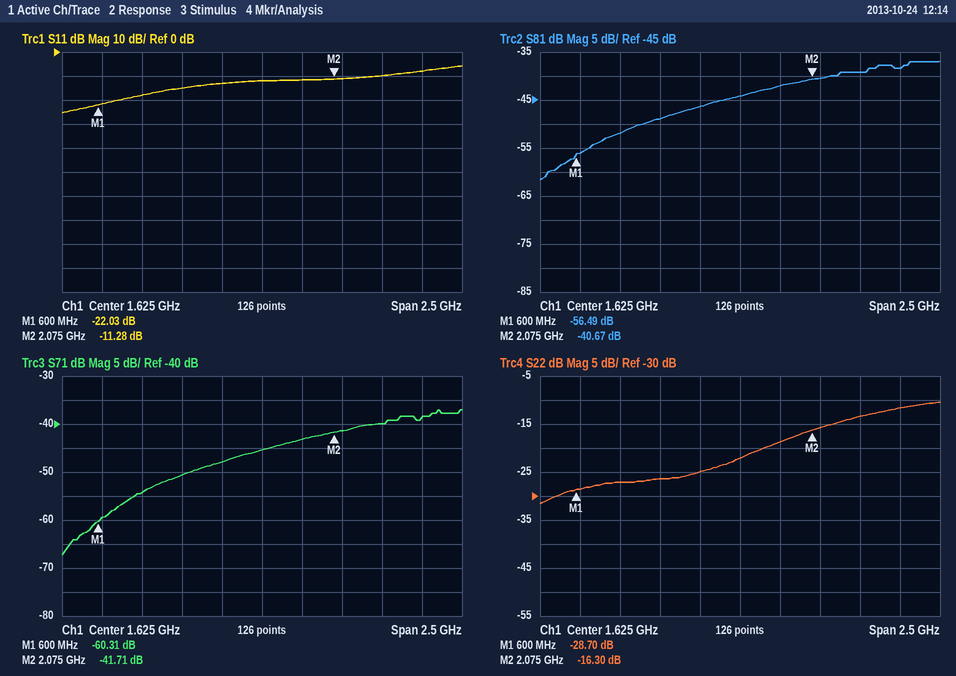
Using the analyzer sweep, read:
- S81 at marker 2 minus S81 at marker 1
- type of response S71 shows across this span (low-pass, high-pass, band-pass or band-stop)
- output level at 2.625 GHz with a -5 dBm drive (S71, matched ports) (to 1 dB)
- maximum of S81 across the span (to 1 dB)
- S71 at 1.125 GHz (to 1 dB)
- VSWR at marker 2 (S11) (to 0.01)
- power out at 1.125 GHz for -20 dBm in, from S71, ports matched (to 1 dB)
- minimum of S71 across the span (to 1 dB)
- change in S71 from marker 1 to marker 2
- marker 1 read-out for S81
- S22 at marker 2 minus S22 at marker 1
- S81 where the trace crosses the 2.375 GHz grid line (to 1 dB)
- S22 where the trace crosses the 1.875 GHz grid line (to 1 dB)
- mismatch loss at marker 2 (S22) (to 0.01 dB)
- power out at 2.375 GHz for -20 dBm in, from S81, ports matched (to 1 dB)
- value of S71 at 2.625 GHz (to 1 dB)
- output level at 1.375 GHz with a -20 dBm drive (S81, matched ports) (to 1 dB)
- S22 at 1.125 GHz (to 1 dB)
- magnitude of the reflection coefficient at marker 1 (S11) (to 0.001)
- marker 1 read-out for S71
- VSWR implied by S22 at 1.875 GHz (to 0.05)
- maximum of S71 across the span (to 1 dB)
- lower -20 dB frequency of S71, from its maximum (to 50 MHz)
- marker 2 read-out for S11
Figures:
15.82 dB
high-pass
-44 dBm
-37 dB
-51 dB
1.75
-71 dBm
-67 dB
18.60 dB
-56.49 dB
12.40 dB
-39 dB
-19 dB
0.10 dB
-59 dBm
-39 dB
-66 dBm
-26 dB
0.079
-60.31 dB
1.25
-37 dB
750 MHz
-11.28 dB
